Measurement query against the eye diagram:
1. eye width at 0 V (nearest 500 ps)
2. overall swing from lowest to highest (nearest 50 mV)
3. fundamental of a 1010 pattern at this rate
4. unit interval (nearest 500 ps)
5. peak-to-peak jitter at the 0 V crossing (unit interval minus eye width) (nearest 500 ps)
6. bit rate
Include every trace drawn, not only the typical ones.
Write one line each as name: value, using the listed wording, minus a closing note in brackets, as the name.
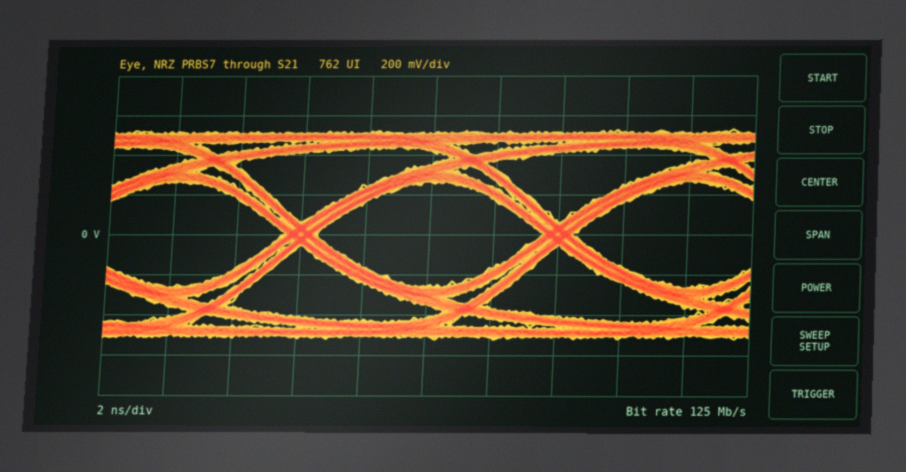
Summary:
eye width at 0 V: 7.0 ns
overall swing from lowest to highest: 1.05 V
fundamental of a 1010 pattern at this rate: 62.5 MHz
unit interval: 8.0 ns
peak-to-peak jitter at the 0 V crossing (unit interval minus eye width): 1.0 ns
bit rate: 125 Mb/s
